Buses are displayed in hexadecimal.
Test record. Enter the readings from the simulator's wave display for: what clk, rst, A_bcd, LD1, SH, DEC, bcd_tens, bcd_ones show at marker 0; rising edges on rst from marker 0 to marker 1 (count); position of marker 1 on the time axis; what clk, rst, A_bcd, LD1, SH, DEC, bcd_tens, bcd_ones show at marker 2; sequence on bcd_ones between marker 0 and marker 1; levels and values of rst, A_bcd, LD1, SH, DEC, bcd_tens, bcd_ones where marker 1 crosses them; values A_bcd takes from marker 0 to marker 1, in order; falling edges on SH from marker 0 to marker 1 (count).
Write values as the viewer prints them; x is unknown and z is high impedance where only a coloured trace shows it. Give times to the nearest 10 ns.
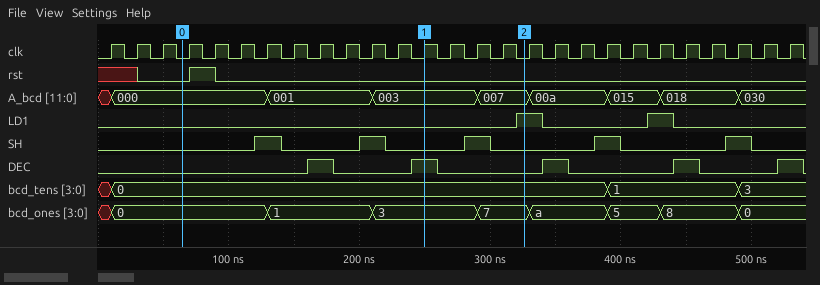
clk=0, rst=0, A_bcd=000, LD1=0, SH=0, DEC=0, bcd_tens=0, bcd_ones=0
1
250 ns
clk=0, rst=0, A_bcd=007, LD1=1, SH=0, DEC=0, bcd_tens=0, bcd_ones=7
0, 1, 3
rst=0, A_bcd=003, LD1=0, SH=0, DEC=1, bcd_tens=0, bcd_ones=3
000, 001, 003
2
